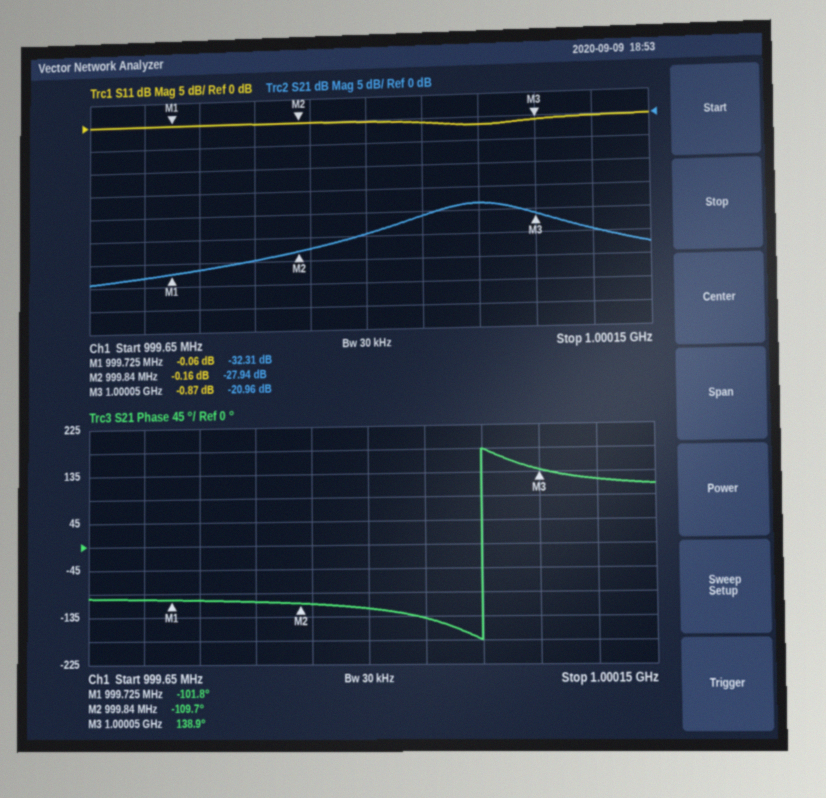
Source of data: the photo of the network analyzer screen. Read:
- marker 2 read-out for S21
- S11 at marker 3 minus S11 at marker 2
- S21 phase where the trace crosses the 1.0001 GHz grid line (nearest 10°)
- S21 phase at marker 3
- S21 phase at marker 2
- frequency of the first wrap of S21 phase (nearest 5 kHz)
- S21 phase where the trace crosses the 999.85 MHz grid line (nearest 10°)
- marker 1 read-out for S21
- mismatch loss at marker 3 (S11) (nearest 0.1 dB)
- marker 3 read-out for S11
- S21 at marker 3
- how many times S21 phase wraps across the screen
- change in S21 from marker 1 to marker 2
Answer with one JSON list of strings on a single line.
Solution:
["-27.94 dB", "-0.71 dB", "120°", "138.9°", "-109.7°", "1.000000 GHz", "-110°", "-32.31 dB", "7.4 dB", "-0.87 dB", "-20.96 dB", "1", "4.37 dB"]
